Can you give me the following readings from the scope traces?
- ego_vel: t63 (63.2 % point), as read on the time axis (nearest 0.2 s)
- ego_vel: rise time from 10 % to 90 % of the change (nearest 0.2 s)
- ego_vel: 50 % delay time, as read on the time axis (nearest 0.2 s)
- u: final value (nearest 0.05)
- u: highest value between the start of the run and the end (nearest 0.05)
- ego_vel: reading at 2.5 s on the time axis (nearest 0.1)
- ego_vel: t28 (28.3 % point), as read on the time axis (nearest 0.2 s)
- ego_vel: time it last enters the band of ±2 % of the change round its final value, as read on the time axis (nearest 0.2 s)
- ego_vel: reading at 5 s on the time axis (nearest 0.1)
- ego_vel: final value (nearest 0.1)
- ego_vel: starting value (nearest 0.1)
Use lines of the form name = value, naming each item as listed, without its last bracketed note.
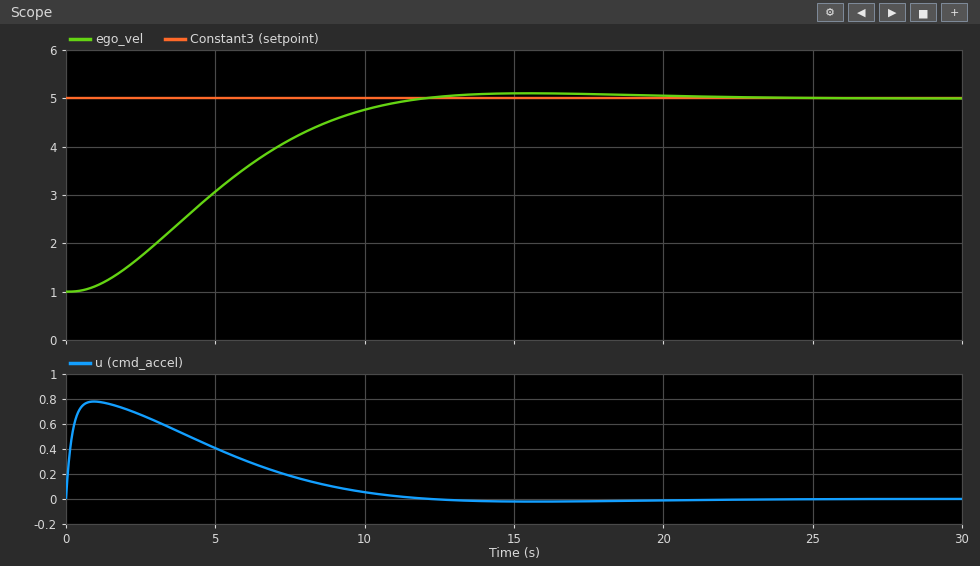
ego_vel: t63 (63.2 % point), as read on the time axis = 6.0 s
ego_vel: rise time from 10 % to 90 % of the change = 7.4 s
ego_vel: 50 % delay time, as read on the time axis = 4.8 s
u: final value = 0.00
u: highest value between the start of the run and the end = 0.80
ego_vel: reading at 2.5 s on the time axis = 1.7
ego_vel: t28 (28.3 % point), as read on the time axis = 3.2 s
ego_vel: time it last enters the band of ±2 % of the change round its final value, as read on the time axis = 18.2 s
ego_vel: reading at 5 s on the time axis = 3.1
ego_vel: final value = 5.0
ego_vel: starting value = 1.0
